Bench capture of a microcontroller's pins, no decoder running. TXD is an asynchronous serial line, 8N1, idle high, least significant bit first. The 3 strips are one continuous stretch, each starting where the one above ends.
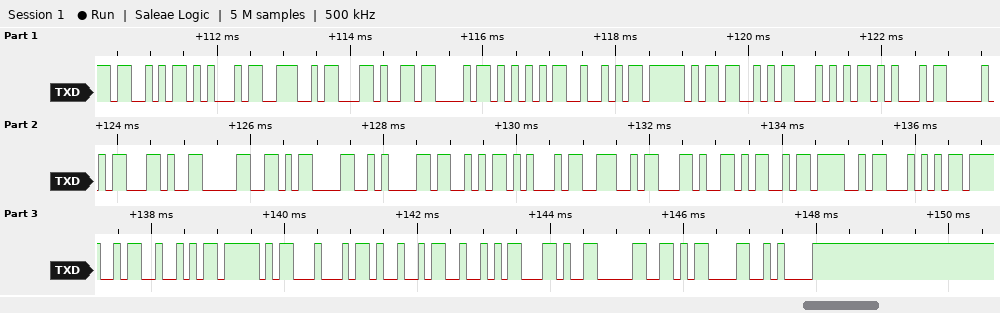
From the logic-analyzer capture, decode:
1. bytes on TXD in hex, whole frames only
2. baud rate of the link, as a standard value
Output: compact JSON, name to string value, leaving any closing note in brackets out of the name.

{"bytes on TXD in hex, whole frames only": "0x53 0x45 0x4E 0x2C 0x43 0x55 0x52 0x5F 0x53 0x54 0x45 0x50 0x2C 0x30 0x0D 0x0A 0x53 0x45 0x4E 0x2C 0x4D 0x4F 0x54 0x4F 0x52 0x5F 0x44 0x49 0x52 0x2C 0x30 0x0D 0x0A", "baud rate of the link, as a standard value": "9600 baud"}
